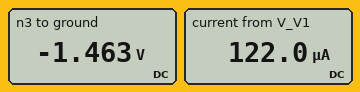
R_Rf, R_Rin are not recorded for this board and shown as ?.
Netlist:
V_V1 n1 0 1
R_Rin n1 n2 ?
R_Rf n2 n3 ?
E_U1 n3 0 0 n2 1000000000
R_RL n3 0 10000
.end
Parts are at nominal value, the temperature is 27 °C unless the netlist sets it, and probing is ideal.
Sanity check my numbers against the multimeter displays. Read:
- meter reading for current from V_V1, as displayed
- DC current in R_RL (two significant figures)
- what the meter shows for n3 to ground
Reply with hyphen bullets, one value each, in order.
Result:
- 122.0 µA
- 150 µA
- -1.463 V
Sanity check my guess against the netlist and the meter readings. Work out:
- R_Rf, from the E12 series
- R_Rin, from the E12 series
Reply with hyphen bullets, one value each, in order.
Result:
- 12 kΩ
- 8.2 kΩ
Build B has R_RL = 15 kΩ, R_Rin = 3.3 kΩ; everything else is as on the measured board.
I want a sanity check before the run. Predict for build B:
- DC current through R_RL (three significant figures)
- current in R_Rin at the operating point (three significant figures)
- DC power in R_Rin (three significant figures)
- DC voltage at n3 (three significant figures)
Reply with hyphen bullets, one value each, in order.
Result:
- 242 µA
- 303 µA
- 303 µW
- -3.64 V
